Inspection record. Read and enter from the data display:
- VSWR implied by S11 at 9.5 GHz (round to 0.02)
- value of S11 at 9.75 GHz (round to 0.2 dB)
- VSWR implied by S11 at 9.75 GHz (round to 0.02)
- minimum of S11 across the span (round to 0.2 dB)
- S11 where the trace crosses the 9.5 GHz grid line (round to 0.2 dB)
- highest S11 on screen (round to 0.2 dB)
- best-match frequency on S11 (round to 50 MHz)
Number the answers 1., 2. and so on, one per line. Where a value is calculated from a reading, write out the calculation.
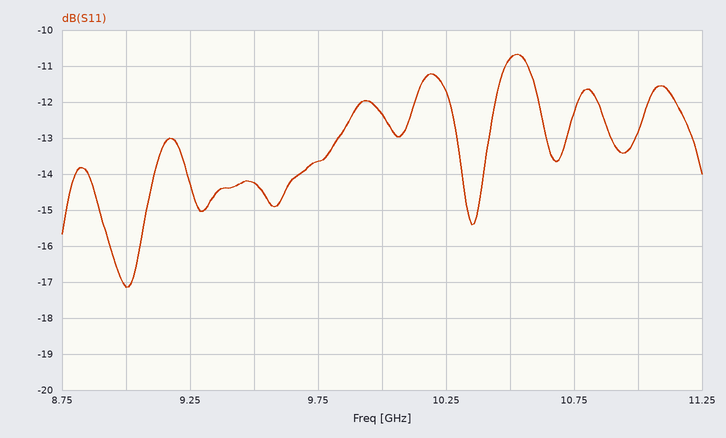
1. |Γ| = 10^(-14.2/20) = 0.1950; VSWR = (1 + 0.1950)/(1 − 0.1950) ≈ 1.48
2. -13.6 dB
3. |Γ| = 10^(-13.6/20) = 0.2089; VSWR = (1 + 0.2089)/(1 − 0.2089) ≈ 1.53, so 1.52 to the nearest 0.02
4. -17.2 dB
5. -14.2 dB
6. -10.6 dB
7. 9.00 GHz
